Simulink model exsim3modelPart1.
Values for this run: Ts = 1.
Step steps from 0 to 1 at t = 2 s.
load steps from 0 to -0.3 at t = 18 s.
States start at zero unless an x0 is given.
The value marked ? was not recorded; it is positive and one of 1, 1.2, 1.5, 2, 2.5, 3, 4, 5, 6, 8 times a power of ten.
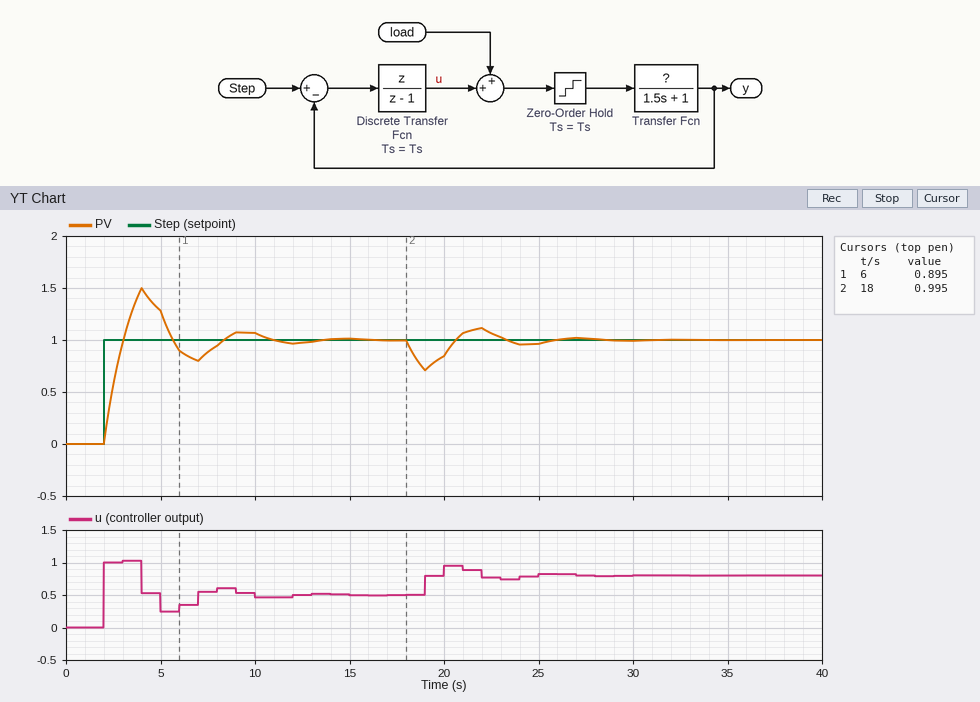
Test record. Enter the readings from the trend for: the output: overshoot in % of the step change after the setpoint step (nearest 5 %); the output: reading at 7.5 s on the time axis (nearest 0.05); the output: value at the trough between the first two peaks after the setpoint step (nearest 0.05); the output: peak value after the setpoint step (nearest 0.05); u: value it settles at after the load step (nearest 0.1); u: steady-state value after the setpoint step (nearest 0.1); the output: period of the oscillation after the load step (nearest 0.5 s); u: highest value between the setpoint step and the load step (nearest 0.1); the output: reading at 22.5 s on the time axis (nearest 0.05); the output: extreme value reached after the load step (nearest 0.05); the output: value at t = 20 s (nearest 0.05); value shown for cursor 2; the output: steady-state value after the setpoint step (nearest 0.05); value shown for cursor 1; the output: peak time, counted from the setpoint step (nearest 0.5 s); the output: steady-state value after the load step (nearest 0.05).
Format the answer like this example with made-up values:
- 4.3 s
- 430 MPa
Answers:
- 50 %
- 0.90
- 0.80
- 1.50
- 0.8
- 0.5
- 5.0 s
- 1.0
- 1.05
- 0.70
- 0.85
- 0.995
- 1.00
- 0.895
- 2.0 s
- 1.00
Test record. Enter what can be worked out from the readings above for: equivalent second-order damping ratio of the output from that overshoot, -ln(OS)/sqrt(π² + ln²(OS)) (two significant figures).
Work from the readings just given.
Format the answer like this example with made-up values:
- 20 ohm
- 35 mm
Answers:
- 0.22
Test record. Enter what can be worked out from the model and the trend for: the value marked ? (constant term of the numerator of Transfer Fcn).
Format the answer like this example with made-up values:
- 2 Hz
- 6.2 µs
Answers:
- 2
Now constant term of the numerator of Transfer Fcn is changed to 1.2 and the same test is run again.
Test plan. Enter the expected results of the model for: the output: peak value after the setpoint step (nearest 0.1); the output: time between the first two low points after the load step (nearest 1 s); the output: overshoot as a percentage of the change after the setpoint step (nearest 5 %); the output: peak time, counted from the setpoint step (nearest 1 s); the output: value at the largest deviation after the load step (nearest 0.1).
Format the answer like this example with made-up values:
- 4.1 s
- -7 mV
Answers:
- 1.3
- 8 s
- 35 %
- 3 s
- 0.8
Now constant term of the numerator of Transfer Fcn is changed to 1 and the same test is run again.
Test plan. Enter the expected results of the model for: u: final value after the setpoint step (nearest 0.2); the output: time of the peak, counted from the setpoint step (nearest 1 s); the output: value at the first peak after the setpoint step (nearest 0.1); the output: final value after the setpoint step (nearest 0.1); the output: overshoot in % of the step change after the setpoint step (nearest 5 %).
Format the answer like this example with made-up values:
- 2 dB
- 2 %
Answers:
- 1.0
- 4 s
- 1.3
- 1.0
- 25 %
